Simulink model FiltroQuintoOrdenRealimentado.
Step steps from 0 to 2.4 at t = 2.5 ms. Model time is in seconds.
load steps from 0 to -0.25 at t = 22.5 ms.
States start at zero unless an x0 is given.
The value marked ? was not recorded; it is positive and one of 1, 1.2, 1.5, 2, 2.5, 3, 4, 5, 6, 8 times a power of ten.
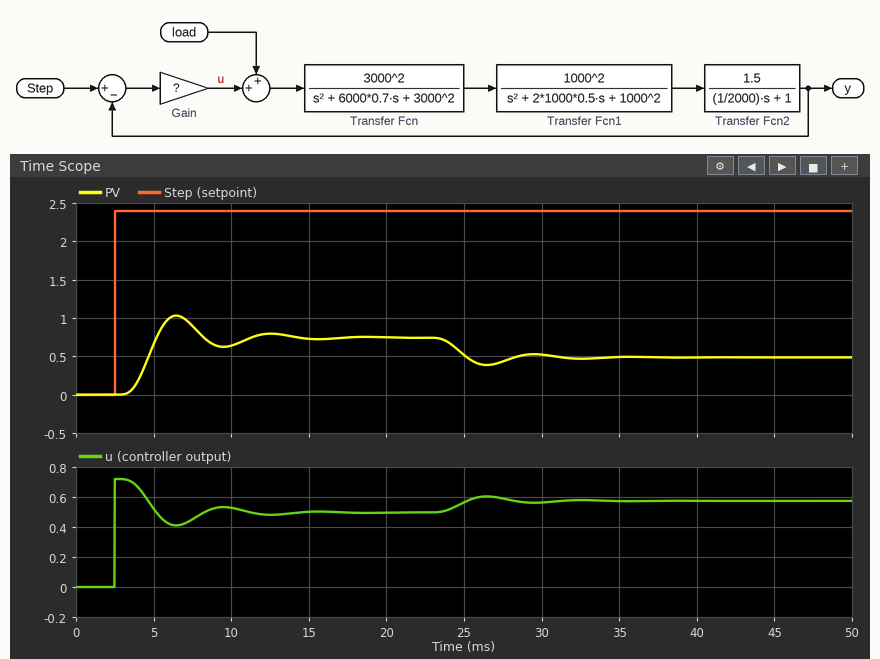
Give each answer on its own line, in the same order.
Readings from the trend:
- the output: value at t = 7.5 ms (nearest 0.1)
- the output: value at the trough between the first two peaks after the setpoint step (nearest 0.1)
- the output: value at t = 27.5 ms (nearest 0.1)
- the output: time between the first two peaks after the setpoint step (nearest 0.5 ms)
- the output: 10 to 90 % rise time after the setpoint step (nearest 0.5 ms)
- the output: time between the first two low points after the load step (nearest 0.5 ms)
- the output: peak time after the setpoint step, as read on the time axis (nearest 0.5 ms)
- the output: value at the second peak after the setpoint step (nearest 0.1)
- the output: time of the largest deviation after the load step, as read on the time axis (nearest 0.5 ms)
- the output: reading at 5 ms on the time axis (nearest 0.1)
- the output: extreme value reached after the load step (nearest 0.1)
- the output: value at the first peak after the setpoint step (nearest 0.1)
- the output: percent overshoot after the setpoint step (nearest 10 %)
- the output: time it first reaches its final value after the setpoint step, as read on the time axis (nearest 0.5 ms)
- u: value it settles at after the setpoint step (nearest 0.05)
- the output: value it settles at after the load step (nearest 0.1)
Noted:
0.9
0.6
0.4
6.0 ms
1.5 ms
6.0 ms
6.5 ms
0.8
26.5 ms
0.7
0.4
1.0
40 %
5.0 ms
0.50
0.5
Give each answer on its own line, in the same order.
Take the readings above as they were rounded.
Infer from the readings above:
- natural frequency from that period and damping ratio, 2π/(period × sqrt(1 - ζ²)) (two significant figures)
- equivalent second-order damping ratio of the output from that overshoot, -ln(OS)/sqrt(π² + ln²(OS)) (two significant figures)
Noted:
1.1 rad/ms
0.28
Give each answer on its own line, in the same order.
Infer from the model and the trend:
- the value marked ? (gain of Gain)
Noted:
0.3
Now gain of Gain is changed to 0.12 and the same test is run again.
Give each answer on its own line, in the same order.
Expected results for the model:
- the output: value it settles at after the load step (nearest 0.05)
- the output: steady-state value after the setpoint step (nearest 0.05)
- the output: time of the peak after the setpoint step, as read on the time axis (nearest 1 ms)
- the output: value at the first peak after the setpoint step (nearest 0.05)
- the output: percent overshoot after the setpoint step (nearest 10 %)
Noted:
0.05
0.35
7 ms
0.45
20 %
